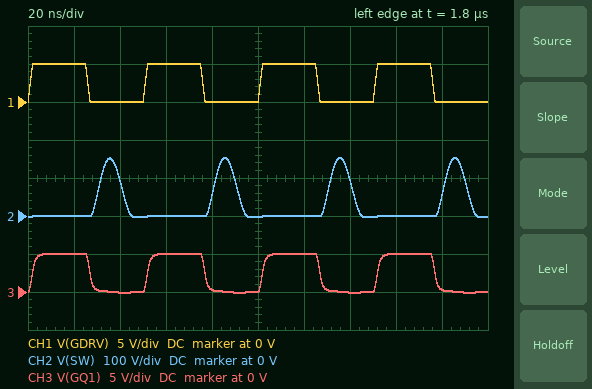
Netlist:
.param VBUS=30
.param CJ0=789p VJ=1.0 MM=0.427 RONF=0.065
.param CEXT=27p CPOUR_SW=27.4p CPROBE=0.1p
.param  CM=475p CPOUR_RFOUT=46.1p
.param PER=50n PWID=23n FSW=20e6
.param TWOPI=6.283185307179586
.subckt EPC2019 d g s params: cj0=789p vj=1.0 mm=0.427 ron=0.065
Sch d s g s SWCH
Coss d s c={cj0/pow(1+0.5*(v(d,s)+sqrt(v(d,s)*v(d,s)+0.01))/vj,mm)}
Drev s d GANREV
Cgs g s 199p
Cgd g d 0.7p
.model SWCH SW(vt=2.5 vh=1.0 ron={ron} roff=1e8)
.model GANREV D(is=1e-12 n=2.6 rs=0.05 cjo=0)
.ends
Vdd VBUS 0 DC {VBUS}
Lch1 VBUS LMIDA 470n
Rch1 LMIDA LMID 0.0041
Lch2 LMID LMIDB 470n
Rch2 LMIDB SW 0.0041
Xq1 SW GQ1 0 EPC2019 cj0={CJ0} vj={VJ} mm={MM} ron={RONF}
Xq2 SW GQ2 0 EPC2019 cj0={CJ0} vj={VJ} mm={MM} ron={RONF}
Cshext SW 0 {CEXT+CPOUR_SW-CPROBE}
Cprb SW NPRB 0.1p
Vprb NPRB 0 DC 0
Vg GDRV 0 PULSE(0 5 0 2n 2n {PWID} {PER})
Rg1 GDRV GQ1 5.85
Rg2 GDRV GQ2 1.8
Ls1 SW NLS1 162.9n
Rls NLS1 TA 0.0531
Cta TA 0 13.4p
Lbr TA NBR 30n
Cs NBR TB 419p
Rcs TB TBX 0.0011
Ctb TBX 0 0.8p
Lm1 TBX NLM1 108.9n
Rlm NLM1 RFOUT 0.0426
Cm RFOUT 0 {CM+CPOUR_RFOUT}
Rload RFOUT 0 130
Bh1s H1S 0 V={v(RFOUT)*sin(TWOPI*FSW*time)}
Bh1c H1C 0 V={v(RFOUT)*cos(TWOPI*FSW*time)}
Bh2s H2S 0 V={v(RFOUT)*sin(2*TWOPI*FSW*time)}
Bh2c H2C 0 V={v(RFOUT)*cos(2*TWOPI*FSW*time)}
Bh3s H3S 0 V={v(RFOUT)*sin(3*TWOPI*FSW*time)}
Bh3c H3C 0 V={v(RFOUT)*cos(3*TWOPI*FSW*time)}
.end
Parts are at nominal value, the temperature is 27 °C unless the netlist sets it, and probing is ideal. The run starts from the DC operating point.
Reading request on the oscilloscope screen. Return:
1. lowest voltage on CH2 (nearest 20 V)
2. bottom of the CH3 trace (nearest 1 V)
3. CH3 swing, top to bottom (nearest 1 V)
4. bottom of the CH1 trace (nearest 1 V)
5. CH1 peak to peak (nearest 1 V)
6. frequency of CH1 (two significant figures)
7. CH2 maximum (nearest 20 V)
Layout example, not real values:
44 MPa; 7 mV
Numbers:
0 V; 0 V; 5 V; 0 V; 5 V; 20 MHz; 160 V
